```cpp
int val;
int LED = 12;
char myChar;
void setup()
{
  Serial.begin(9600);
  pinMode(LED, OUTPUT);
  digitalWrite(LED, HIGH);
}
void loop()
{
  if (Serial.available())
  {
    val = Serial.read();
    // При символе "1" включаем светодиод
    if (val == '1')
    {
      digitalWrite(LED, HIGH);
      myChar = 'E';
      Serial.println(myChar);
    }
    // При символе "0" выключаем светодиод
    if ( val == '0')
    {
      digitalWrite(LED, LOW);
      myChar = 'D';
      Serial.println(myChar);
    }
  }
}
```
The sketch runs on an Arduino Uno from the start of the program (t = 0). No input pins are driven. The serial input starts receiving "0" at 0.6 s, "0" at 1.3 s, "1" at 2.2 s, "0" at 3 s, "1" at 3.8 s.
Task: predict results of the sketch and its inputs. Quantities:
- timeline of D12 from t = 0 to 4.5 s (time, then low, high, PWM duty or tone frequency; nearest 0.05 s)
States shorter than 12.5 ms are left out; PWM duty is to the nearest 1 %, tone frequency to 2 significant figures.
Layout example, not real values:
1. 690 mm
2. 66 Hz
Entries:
1. 0 s high; 0.6 s low; 2.2 s high; 3 s low; 3.8 s high
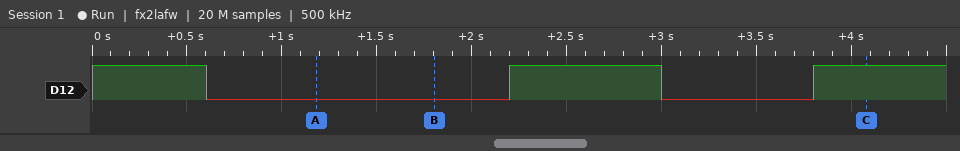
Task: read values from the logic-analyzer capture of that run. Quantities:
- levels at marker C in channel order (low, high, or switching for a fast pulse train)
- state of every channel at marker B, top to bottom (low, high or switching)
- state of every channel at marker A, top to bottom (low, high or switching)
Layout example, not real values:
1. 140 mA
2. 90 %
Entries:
1. D12 high
2. D12 low
3. D12 low
